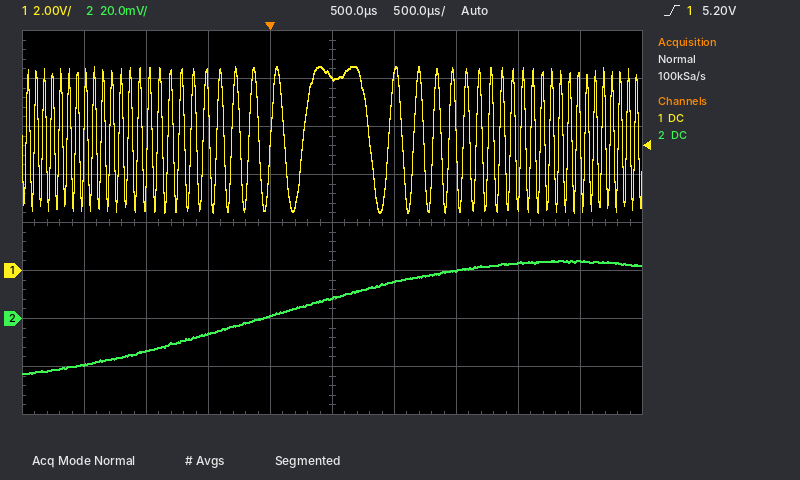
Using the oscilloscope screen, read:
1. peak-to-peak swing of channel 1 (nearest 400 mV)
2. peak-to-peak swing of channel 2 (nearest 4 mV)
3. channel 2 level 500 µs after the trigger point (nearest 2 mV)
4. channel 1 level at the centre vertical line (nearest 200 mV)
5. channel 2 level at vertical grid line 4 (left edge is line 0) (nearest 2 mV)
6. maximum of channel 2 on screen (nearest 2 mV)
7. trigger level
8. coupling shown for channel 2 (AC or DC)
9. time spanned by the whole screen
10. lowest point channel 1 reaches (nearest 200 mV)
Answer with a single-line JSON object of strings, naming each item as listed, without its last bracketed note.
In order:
{"peak-to-peak swing of channel 1": "6.0 V", "peak-to-peak swing of channel 2": "48 mV", "channel 2 level 500 µs after the trigger point": "8 mV", "channel 1 level at the centre vertical line": "8.0 V", "channel 2 level at vertical grid line 4 (left edge is line 0)": "2 mV", "maximum of channel 2 on screen": "24 mV", "trigger level": "5.20 V", "coupling shown for channel 2": "DC", "time spanned by the whole screen": "5 ms", "lowest point channel 1 reaches": "2.4 V"}
